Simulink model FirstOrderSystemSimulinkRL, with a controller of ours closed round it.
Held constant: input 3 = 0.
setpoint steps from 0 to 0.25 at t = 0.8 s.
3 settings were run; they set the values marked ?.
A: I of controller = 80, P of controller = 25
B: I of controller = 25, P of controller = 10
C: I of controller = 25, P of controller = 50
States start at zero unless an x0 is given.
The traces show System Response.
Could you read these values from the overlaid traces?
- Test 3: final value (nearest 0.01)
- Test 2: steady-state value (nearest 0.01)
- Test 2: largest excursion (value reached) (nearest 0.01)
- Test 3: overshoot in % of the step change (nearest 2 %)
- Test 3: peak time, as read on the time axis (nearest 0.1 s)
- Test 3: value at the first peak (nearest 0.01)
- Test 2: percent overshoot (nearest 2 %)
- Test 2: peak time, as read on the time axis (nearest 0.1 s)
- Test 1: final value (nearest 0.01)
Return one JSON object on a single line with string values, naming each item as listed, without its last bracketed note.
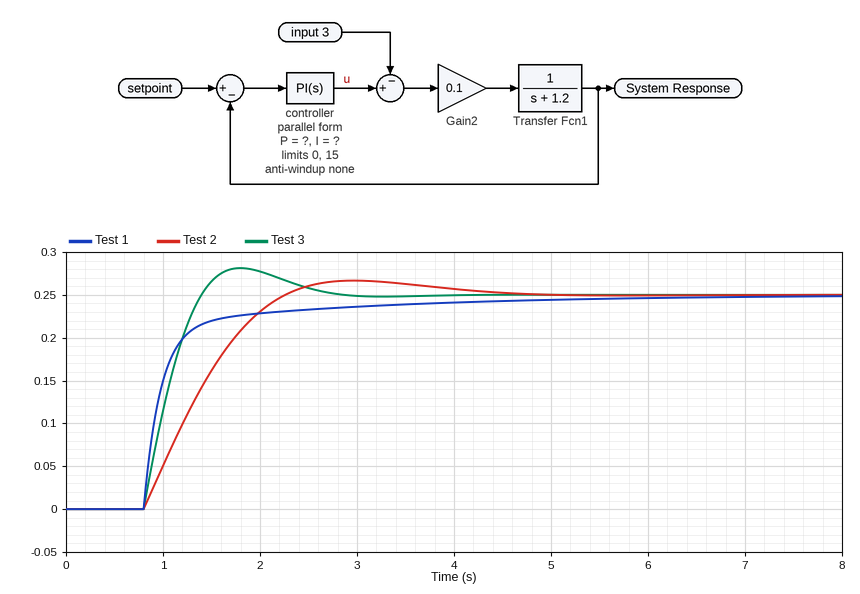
{"Test 3: final value": "0.25", "Test 2: steady-state value": "0.25", "Test 2: largest excursion (value reached)": "0.27", "Test 3: overshoot in % of the step change": "12 %", "Test 3: peak time, as read on the time axis": "1.8 s", "Test 3: value at the first peak": "0.28", "Test 2: percent overshoot": "6 %", "Test 2: peak time, as read on the time axis": "3.0 s", "Test 1: final value": "0.25"}
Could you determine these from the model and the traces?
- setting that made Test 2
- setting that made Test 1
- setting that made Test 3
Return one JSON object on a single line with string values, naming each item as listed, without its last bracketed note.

{"setting that made Test 2": "B", "setting that made Test 1": "C", "setting that made Test 3": "A"}
